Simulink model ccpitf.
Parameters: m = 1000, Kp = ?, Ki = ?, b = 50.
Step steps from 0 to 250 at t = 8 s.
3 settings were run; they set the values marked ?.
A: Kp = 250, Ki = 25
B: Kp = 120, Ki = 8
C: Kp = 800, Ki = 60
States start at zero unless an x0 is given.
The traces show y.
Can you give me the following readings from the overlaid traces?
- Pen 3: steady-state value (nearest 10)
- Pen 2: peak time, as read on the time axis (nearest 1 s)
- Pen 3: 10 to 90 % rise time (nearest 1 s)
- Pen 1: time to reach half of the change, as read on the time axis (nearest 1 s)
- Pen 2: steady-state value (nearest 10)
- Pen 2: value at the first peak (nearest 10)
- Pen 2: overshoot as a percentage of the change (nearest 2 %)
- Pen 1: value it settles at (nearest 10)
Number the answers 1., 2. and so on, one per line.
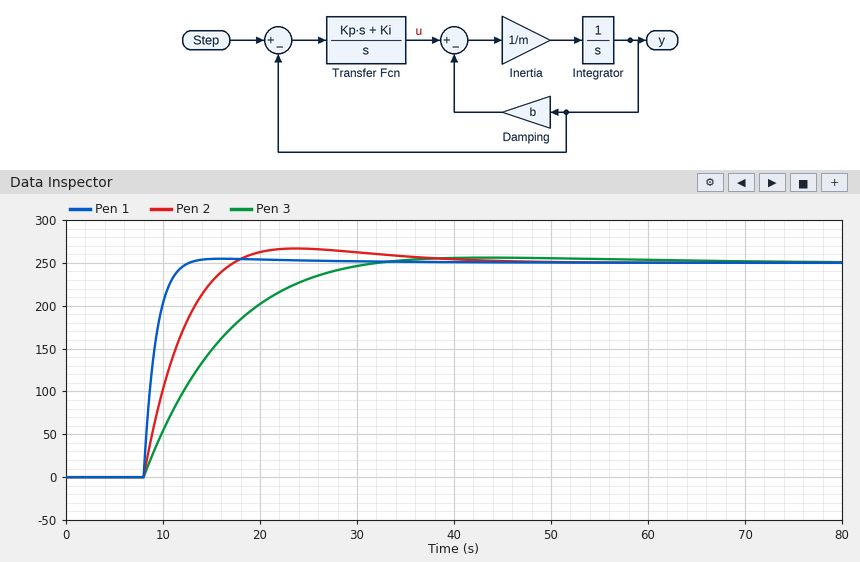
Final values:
1. 250
2. 24 s
3. 15 s
4. 9 s
5. 250
6. 270
7. 6 %
8. 250
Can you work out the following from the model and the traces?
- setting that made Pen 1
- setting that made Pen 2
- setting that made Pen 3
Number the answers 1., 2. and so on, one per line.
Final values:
1. C
2. A
3. B
